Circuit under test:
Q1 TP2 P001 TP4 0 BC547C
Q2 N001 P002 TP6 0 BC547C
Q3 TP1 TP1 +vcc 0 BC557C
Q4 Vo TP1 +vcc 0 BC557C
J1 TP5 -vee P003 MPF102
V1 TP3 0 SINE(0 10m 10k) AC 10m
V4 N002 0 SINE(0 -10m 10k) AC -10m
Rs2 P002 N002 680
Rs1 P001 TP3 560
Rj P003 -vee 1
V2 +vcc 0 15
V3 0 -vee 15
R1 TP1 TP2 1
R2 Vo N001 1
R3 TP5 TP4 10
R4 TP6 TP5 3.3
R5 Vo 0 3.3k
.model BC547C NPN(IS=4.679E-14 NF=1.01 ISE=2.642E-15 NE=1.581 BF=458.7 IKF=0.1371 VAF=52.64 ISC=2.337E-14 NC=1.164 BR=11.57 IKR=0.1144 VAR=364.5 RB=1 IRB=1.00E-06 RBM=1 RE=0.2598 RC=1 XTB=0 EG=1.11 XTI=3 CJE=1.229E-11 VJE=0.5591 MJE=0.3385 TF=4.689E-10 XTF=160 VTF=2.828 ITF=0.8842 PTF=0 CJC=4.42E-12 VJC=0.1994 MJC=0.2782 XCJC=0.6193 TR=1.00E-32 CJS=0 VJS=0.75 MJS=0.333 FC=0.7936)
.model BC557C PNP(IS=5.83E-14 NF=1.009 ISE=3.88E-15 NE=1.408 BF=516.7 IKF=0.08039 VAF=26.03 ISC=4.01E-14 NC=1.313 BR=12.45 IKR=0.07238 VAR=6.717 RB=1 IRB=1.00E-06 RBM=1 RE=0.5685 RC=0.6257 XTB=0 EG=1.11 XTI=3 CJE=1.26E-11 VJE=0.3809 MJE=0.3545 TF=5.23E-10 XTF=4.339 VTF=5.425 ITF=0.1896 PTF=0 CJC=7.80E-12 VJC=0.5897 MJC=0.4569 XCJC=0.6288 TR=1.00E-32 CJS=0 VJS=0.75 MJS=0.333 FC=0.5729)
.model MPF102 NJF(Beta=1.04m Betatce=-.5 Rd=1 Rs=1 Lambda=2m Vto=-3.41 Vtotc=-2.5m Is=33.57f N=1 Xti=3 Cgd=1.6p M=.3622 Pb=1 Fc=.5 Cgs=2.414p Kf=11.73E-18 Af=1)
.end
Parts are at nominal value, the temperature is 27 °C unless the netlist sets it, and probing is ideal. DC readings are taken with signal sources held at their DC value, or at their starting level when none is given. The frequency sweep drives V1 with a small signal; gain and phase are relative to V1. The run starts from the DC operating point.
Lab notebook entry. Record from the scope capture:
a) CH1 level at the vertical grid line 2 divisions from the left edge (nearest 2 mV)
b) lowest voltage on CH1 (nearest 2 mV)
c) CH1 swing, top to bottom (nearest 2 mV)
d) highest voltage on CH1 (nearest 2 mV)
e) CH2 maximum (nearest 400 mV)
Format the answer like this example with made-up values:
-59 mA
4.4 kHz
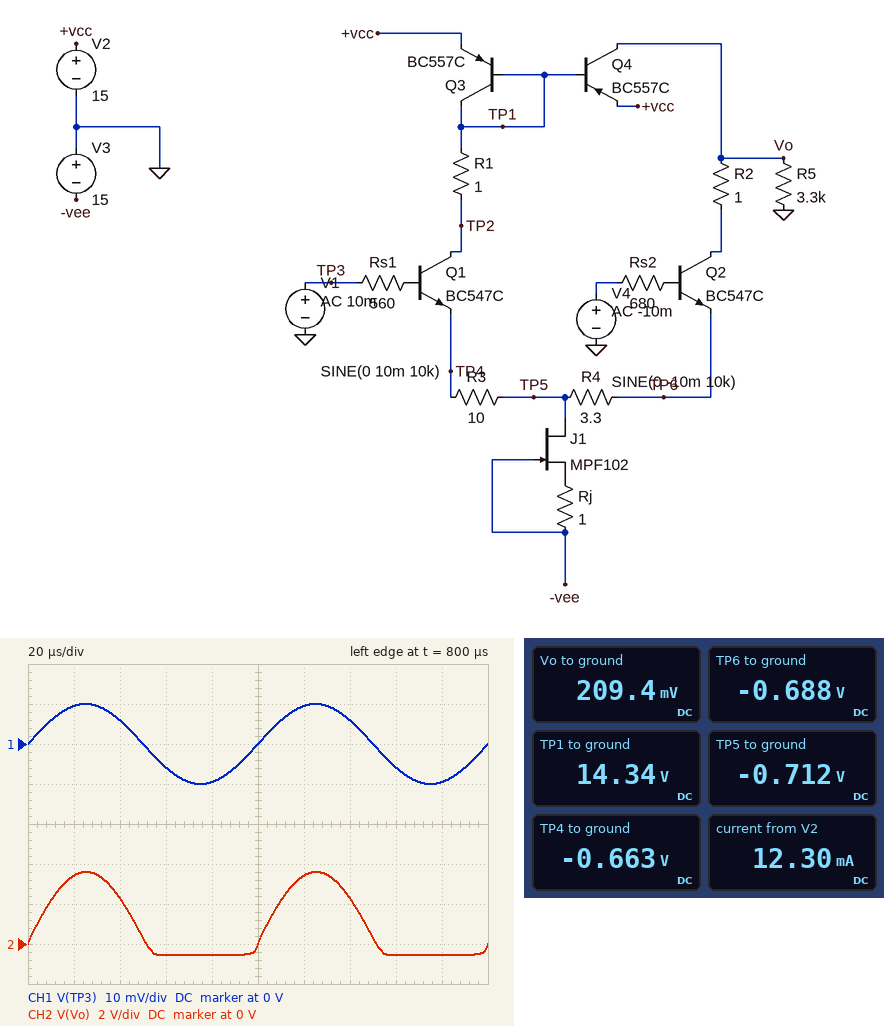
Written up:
6 mV
-10 mV
20 mV
10 mV
3.6 V
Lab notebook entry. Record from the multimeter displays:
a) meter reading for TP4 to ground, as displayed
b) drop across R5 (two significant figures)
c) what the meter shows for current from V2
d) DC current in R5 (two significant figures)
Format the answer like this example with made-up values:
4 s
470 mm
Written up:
-0.663 V
210 mV
12.30 mA
63 µA
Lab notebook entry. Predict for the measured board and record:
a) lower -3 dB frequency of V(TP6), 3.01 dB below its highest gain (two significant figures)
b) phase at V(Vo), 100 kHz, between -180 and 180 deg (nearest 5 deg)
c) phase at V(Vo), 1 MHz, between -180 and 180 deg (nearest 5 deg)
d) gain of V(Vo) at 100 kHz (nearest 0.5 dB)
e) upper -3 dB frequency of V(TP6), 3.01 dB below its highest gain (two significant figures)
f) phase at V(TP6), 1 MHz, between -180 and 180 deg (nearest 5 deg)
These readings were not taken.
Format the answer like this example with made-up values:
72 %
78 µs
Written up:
290 kHz
-15 deg
-70 deg
44.5 dB
110 MHz
10 deg
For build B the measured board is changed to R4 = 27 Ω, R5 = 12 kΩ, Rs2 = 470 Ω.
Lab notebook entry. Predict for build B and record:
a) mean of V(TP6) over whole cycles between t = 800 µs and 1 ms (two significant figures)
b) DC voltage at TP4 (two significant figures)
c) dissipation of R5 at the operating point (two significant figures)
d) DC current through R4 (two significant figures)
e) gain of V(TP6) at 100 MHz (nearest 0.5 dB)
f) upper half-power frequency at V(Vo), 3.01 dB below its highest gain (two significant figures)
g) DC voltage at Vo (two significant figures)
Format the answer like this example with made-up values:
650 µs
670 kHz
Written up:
-660 mV
-680 mV
19 mW
4.0 mA
-7.5 dB
11 MHz
15 V
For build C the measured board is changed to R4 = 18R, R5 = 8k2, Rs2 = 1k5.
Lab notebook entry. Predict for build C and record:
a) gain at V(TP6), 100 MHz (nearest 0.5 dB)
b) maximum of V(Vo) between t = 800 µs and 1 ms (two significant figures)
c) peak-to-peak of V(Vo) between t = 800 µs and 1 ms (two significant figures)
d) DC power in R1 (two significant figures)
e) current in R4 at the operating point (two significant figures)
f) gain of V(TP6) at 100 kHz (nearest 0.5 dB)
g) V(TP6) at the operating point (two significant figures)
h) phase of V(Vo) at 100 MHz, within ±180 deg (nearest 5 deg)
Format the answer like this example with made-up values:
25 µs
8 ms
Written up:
-4.5 dB
15 V
320 mV
57 µW
4.7 mA
-14.0 dB
-670 mV
-110 deg
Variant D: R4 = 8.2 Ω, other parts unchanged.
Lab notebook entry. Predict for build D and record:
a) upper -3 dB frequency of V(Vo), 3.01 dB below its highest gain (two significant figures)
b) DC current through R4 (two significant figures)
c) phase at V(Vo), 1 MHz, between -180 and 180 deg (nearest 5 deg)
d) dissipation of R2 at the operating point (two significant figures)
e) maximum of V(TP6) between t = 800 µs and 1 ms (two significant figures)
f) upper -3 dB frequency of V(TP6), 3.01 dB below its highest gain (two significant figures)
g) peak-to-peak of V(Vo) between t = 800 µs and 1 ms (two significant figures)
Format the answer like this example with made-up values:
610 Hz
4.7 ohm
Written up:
800 kHz
6.3 mA
-50 deg
39 µW
-670 mV
98 MHz
5.4 V
